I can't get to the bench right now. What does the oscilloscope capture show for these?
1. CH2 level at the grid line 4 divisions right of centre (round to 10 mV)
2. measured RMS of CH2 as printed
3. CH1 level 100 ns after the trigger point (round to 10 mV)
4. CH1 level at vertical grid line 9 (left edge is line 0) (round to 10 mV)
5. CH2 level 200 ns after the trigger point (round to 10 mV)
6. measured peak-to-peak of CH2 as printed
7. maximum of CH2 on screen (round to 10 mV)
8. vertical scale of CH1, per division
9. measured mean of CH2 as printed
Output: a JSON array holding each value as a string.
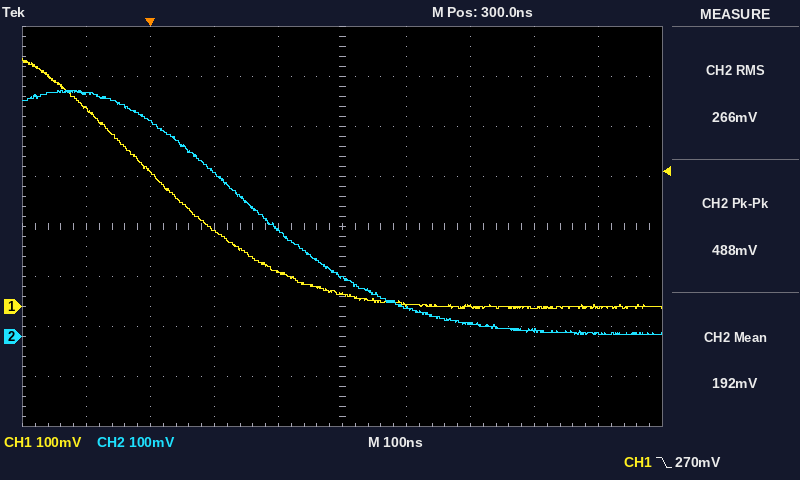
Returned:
["10 mV", "266 mV", "150 mV", "0 mV", "210 mV", "488 mV", "490 mV", "100 mV", "192 mV"]
